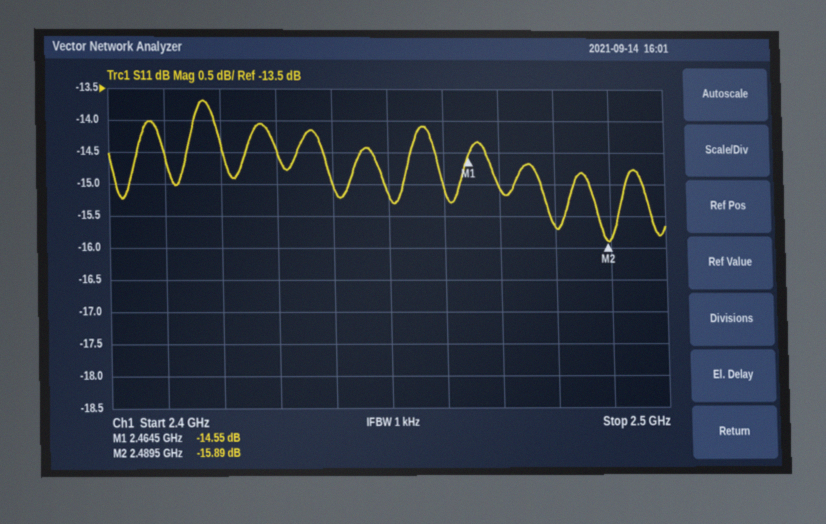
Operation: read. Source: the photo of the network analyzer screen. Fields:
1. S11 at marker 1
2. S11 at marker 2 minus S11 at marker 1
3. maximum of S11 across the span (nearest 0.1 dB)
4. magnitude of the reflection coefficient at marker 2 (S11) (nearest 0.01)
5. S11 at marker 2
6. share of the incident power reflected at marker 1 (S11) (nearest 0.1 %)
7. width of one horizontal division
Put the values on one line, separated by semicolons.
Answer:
-14.55 dB; -1.34 dB; -13.7 dB; 0.16; -15.89 dB; 3.5 %; 10 MHz
